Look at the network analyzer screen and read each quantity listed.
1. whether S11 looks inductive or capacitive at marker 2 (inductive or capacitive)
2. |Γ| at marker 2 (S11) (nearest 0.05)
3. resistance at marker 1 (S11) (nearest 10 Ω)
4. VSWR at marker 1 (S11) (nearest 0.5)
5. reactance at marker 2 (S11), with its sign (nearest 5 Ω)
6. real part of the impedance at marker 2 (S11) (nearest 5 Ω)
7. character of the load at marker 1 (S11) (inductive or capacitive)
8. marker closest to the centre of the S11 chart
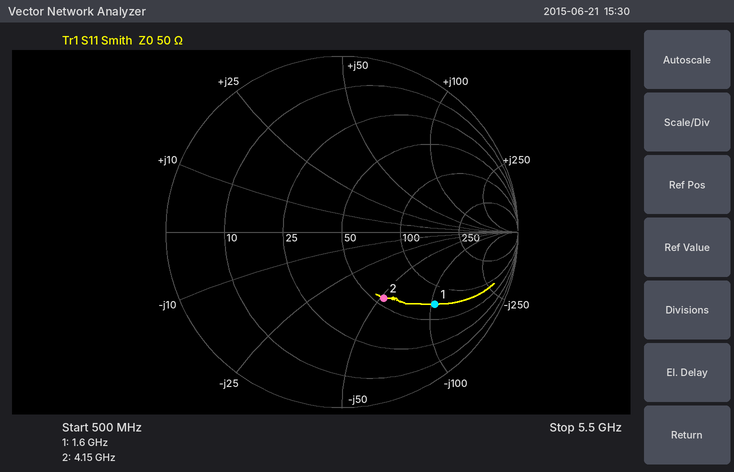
capacitive
0.45
70 Ω
5.0
-50 Ω
55 Ω
capacitive
marker 2
